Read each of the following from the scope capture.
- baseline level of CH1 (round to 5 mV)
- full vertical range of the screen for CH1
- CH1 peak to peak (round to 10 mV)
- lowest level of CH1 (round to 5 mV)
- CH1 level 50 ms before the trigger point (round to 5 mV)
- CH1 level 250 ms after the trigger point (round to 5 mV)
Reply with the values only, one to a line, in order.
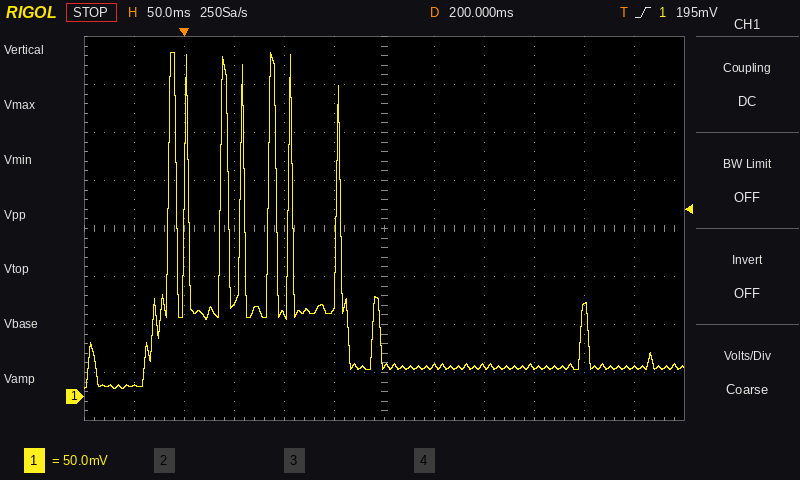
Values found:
30 mV
400 mV
350 mV
10 mV
10 mV
30 mV
